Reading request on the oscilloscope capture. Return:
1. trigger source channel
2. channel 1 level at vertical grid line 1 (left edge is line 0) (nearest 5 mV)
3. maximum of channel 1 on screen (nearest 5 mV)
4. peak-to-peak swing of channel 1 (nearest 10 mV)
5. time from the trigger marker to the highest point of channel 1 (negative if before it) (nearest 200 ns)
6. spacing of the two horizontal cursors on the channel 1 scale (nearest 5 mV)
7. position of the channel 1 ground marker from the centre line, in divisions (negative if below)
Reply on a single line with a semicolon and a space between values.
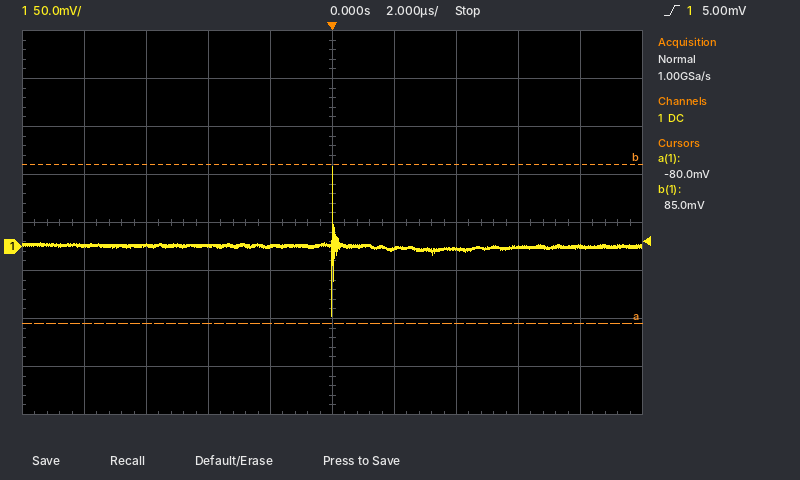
channel 1; 0 mV; 85 mV; 160 mV; 0.0 µs; 165 mV; -0.5 div
